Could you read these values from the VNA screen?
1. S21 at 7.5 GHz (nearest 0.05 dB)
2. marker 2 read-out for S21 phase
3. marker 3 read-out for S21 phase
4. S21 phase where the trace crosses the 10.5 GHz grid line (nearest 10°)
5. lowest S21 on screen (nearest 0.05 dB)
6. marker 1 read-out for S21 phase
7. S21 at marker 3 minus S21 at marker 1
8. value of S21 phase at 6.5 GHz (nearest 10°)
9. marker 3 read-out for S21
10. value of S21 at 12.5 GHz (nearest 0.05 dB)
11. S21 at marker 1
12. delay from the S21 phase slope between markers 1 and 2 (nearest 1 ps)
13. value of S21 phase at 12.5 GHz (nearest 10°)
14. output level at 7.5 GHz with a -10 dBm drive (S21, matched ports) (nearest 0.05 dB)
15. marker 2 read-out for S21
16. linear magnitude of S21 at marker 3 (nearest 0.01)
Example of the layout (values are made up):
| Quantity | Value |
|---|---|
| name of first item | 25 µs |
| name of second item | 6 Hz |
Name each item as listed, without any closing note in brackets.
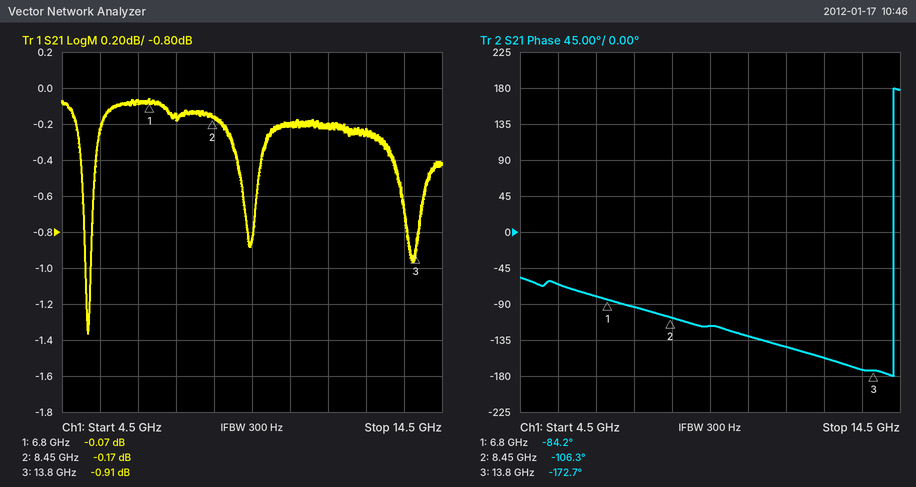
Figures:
| Quantity | Value |
|---|---|
| S21 at 7.5 GHz | -0.15 dB |
| marker 2 read-out for S21 phase | -106.3° |
| marker 3 read-out for S21 phase | -172.7° |
| S21 phase where the trace crosses the 10.5 GHz grid line | -130° |
| lowest S21 on screen | -1.35 dB |
| marker 1 read-out for S21 phase | -84.2° |
| S21 at marker 3 minus S21 at marker 1 | -0.84 dB |
| value of S21 phase at 6.5 GHz | -80° |
| marker 3 read-out for S21 | -0.91 dB |
| value of S21 at 12.5 GHz | -0.25 dB |
| S21 at marker 1 | -0.07 dB |
| delay from the S21 phase slope between markers 1 and 2 | 37 ps |
| value of S21 phase at 12.5 GHz | -160° |
| output level at 7.5 GHz with a -10 dBm drive (S21, matched ports) | -10.15 dBm |
| marker 2 read-out for S21 | -0.17 dB |
| linear magnitude of S21 at marker 3 | 0.90 |
